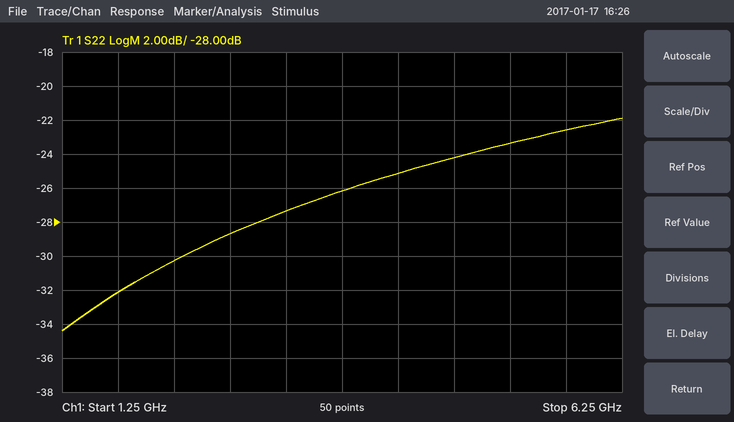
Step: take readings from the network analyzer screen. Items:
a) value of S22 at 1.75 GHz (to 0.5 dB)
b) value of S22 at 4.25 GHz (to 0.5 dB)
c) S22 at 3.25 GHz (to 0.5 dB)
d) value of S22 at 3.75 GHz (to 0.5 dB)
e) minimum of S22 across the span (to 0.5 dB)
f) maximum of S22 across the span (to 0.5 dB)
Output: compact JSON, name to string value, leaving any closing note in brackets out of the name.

{"value of S22 at 1.75 GHz": "-32.0 dB", "value of S22 at 4.25 GHz": "-25.0 dB", "S22 at 3.25 GHz": "-27.5 dB", "value of S22 at 3.75 GHz": "-26.0 dB", "minimum of S22 across the span": "-34.5 dB", "maximum of S22 across the span": "-22.0 dB"}
